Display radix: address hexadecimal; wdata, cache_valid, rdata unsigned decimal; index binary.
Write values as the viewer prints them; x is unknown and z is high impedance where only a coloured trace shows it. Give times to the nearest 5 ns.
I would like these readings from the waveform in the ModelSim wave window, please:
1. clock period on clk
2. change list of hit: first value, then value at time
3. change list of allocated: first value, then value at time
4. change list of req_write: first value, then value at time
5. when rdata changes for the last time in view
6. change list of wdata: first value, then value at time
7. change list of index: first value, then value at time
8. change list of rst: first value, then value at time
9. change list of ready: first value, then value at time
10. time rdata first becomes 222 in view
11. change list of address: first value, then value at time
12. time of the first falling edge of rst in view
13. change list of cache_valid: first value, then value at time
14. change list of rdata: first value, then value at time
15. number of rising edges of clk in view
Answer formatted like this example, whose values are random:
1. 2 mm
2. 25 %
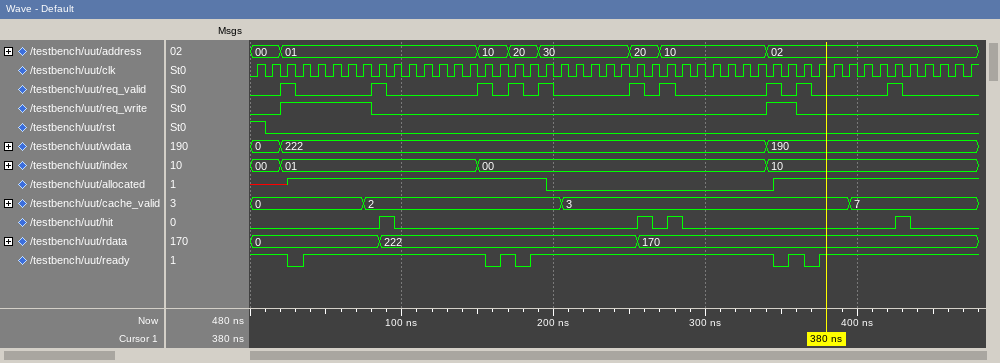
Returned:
1. 10 ns
2. 0, 1 at 85 ns, 0 at 95 ns, 1 at 255 ns, 0 at 265 ns, 1 at 275 ns, 0 at 285 ns, 1 at 425 ns, 0 at 435 ns
3. x, 1 at 25 ns, 0 at 195 ns, 1 at 345 ns
4. 0, 1 at 20 ns, 0 at 80 ns, 1 at 340 ns, 0 at 360 ns
5. 255 ns
6. 0, 222 at 20 ns, 190 at 340 ns
7. 00, 01 at 20 ns, 00 at 150 ns, 10 at 340 ns
8. 1, 0 at 10 ns
9. 1, 0 at 25 ns, 1 at 35 ns, 0 at 155 ns, 1 at 165 ns, 0 at 175 ns, 1 at 185 ns, 0 at 345 ns, 1 at 355 ns, 0 at 365 ns, 1 at 375 ns
10. 85 ns
11. 00, 01 at 20 ns, 10 at 150 ns, 20 at 170 ns, 30 at 190 ns, 20 at 250 ns, 10 at 270 ns, 02 at 340 ns
12. 10 ns
13. 0, 2 at 75 ns, 3 at 205 ns, 7 at 395 ns
14. 0, 222 at 85 ns, 170 at 255 ns
15. 48
